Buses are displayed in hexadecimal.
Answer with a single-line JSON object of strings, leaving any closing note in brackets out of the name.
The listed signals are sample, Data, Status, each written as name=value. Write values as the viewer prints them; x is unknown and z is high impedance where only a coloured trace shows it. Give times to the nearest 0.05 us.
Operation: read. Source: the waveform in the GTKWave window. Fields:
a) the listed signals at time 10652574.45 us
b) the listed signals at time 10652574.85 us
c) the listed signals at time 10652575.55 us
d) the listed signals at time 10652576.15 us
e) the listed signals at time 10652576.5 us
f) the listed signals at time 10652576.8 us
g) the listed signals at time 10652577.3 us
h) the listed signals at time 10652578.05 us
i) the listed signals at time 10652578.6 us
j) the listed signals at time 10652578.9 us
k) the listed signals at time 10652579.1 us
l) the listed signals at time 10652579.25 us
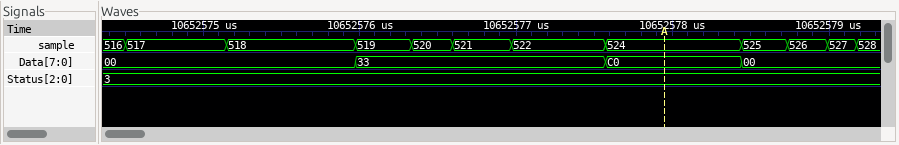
{"the listed signals at time 10652574.45 us": "sample=516, Data=00, Status=3", "the listed signals at time 10652574.85 us": "sample=517, Data=00, Status=3", "the listed signals at time 10652575.55 us": "sample=518, Data=00, Status=3", "the listed signals at time 10652576.15 us": "sample=519, Data=33, Status=3", "the listed signals at time 10652576.5 us": "sample=520, Data=33, Status=3", "the listed signals at time 10652576.8 us": "sample=521, Data=33, Status=3", "the listed signals at time 10652577.3 us": "sample=522, Data=33, Status=3", "the listed signals at time 10652578.05 us": "sample=524, Data=C0, Status=3", "the listed signals at time 10652578.6 us": "sample=525, Data=00, Status=3", "the listed signals at time 10652578.9 us": "sample=526, Data=00, Status=3", "the listed signals at time 10652579.1 us": "sample=527, Data=00, Status=3", "the listed signals at time 10652579.25 us": "sample=528, Data=00, Status=3"}
